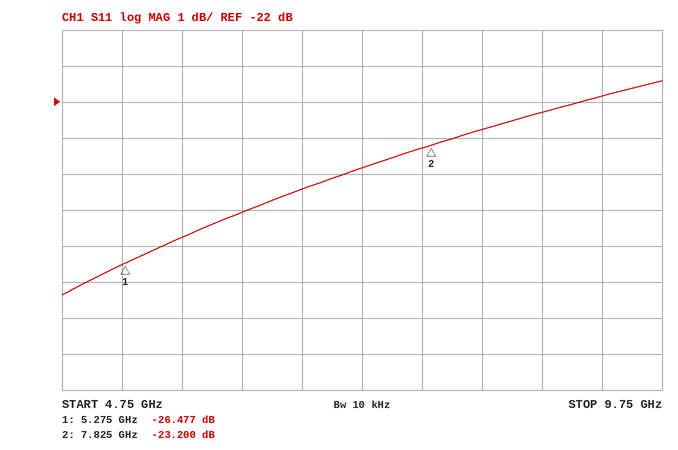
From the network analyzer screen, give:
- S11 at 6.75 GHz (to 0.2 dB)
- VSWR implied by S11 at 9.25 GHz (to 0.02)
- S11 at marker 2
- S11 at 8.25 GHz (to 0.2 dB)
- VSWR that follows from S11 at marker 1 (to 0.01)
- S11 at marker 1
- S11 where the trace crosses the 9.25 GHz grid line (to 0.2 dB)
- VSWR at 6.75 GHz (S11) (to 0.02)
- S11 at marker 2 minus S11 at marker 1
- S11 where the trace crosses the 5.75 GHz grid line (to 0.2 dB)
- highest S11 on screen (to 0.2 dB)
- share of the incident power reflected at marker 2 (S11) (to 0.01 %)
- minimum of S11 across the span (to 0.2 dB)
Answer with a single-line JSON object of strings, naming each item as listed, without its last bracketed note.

{"S11 at 6.75 GHz": "-24.4 dB", "VSWR implied by S11 at 9.25 GHz": "1.18", "S11 at marker 2": "-23.200 dB", "S11 at 8.25 GHz": "-22.8 dB", "VSWR that follows from S11 at marker 1": "1.10", "S11 at marker 1": "-26.477 dB", "S11 where the trace crosses the 9.25 GHz grid line": "-21.8 dB", "VSWR at 6.75 GHz (S11)": "1.12", "S11 at marker 2 minus S11 at marker 1": "3.277 dB", "S11 where the trace crosses the 5.75 GHz grid line": "-25.8 dB", "highest S11 on screen": "-21.4 dB", "share of the incident power reflected at marker 2 (S11)": "0.48 %", "minimum of S11 across the span": "-27.4 dB"}
